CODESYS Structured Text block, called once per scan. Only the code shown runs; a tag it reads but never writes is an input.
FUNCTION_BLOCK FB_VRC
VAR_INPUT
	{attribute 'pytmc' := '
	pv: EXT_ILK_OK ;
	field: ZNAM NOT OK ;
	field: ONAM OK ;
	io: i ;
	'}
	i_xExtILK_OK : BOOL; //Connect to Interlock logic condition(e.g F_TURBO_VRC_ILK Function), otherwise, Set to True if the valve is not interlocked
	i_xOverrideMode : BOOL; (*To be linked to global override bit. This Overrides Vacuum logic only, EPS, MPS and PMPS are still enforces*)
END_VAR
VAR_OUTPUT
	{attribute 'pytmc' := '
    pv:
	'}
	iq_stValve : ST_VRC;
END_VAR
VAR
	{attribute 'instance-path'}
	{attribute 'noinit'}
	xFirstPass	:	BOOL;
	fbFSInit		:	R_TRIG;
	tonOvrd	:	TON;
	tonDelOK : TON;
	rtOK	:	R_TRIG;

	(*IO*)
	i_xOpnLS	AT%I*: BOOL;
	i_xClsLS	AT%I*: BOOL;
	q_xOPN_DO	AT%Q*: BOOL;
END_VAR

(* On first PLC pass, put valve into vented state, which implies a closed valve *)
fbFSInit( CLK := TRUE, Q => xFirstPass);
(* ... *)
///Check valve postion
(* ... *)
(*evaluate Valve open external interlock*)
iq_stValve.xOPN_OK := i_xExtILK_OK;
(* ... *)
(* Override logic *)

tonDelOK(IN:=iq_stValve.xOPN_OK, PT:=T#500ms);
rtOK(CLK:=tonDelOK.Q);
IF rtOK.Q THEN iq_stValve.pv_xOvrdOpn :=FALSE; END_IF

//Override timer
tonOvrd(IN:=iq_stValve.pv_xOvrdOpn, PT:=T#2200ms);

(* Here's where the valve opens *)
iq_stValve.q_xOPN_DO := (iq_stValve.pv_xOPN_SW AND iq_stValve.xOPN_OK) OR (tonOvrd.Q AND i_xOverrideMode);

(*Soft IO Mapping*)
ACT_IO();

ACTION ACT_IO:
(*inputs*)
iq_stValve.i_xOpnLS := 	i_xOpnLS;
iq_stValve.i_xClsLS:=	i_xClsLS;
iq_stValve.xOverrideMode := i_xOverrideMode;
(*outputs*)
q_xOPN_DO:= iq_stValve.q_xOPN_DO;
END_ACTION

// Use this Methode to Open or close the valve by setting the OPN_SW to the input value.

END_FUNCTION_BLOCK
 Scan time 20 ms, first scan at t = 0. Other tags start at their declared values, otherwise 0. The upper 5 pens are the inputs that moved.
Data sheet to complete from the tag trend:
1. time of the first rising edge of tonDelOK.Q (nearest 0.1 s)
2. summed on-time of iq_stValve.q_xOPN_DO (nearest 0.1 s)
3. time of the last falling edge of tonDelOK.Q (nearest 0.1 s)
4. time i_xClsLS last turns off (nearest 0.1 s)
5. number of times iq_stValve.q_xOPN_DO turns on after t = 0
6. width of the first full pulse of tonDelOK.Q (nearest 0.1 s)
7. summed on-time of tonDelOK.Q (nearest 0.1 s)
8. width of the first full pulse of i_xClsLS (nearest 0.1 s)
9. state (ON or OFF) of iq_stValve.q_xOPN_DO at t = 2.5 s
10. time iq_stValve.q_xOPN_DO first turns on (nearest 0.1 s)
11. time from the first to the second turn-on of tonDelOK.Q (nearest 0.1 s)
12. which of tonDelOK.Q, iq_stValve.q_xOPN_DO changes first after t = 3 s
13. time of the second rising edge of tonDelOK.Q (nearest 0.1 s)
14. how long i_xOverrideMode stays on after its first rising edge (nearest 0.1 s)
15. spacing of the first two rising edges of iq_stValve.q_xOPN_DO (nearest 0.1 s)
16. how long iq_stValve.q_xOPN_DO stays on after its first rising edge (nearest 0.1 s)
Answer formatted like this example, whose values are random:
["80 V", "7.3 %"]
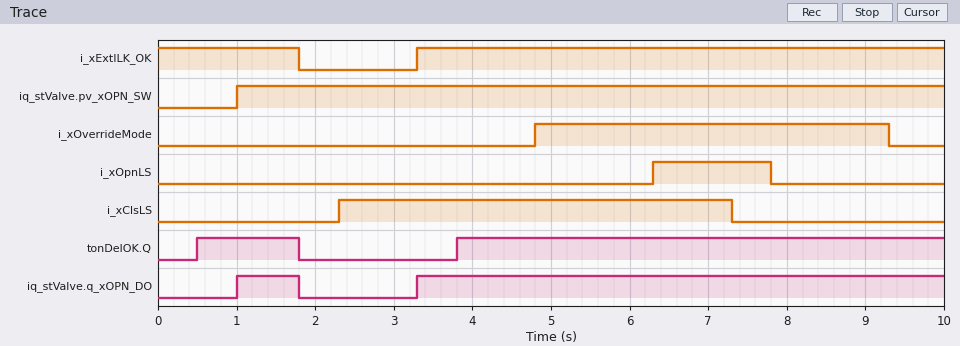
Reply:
["0.5 s", "7.5 s", "1.8 s", "7.3 s", "2", "1.3 s", "7.5 s", "5.0 s", "OFF", "1.0 s", "3.3 s", "iq_stValve.q_xOPN_DO", "3.8 s", "4.5 s", "2.3 s", "0.8 s"]
